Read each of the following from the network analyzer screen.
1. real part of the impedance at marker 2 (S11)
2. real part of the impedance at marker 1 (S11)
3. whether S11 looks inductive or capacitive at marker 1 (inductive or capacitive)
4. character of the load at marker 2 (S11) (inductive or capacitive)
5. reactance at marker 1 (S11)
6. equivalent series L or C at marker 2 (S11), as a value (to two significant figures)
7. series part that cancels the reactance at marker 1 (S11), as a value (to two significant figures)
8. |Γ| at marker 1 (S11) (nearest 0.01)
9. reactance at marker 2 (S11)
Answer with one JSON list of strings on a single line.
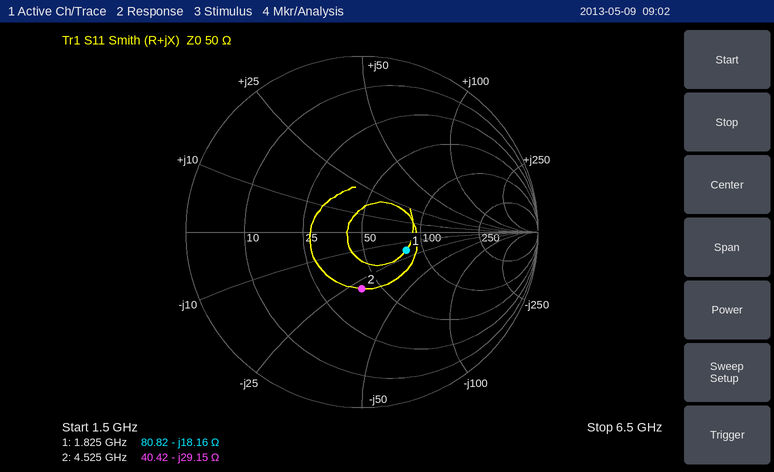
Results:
["40.42 Ω", "80.82 Ω", "capacitive", "capacitive", "-18.16 Ω", "1.2 pF", "1.6 nH", "0.27", "-29.15 Ω"]
